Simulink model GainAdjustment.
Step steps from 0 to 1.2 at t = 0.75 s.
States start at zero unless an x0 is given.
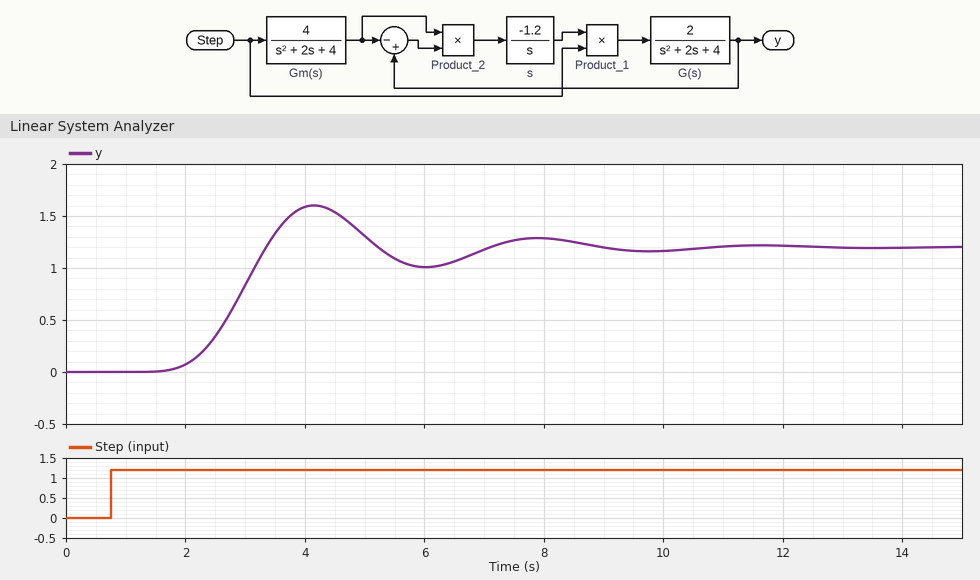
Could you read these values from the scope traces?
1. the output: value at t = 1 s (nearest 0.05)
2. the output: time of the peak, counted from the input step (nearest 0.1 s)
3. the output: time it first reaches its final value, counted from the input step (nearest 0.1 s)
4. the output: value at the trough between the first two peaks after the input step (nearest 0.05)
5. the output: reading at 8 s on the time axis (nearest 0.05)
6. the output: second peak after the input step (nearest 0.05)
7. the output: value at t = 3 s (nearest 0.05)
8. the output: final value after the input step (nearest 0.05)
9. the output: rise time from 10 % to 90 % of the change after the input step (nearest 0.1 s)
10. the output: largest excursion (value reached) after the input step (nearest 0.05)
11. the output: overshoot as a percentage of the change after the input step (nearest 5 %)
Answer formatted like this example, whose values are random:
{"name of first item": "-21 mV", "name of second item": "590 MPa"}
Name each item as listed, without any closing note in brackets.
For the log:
{"the output: value at t = 1 s": "0.00", "the output: time of the peak, counted from the input step": "3.4 s", "the output: time it first reaches its final value, counted from the input step": "2.6 s", "the output: value at the trough between the first two peaks after the input step": "1.00", "the output: reading at 8 s on the time axis": "1.30", "the output: second peak after the input step": "1.30", "the output: value at t = 3 s": "0.85", "the output: final value after the input step": "1.20", "the output: rise time from 10 % to 90 % of the change after the input step": "1.1 s", "the output: largest excursion (value reached) after the input step": "1.60", "the output: overshoot as a percentage of the change after the input step": "35 %"}
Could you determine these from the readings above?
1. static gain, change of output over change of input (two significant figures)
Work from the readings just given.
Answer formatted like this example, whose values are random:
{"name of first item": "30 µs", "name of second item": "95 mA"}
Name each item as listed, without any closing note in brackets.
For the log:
{"static gain, change of output over change of input": "1.0"}
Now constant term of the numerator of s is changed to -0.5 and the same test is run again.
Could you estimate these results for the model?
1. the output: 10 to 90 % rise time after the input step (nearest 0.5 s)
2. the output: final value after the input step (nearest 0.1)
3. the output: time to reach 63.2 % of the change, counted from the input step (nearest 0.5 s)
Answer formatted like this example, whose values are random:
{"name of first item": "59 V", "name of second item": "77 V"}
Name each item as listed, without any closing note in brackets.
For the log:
{"the output: 10 to 90 % rise time after the input step": "4.5 s", "the output: final value after the input step": "1.2", "the output: time to reach 63.2 % of the change, counted from the input step": "3.0 s"}
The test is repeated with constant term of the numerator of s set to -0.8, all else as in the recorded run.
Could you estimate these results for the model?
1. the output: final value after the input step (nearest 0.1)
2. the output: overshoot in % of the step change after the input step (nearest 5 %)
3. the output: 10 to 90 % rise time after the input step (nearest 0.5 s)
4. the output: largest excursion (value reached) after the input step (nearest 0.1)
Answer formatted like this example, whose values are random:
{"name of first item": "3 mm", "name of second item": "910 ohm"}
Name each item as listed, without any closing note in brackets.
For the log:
{"the output: final value after the input step": "1.2", "the output: overshoot in % of the step change after the input step": "10 %", "the output: 10 to 90 % rise time after the input step": "1.5 s", "the output: largest excursion (value reached) after the input step": "1.3"}
